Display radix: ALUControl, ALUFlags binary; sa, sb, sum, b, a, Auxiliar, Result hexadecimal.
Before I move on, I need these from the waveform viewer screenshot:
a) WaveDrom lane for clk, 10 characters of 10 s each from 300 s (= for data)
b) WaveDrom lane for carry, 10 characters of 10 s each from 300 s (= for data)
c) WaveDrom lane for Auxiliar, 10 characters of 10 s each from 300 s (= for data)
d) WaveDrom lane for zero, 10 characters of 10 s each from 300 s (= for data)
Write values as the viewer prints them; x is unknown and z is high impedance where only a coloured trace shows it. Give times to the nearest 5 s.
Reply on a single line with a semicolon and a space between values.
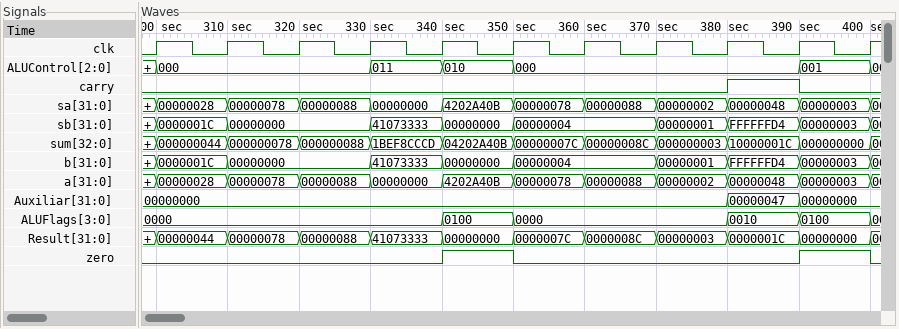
{name: 'clk', wave: 'p.........'}; {name: 'carry', wave: '0.......10'}; {name: 'Auxiliar', wave: '=.......==', data: '00000000 00000047 00000000'}; {name: 'zero', wave: '0...10...1'}
